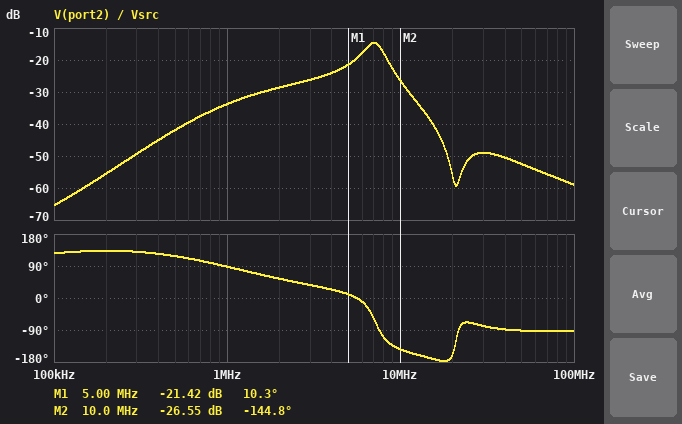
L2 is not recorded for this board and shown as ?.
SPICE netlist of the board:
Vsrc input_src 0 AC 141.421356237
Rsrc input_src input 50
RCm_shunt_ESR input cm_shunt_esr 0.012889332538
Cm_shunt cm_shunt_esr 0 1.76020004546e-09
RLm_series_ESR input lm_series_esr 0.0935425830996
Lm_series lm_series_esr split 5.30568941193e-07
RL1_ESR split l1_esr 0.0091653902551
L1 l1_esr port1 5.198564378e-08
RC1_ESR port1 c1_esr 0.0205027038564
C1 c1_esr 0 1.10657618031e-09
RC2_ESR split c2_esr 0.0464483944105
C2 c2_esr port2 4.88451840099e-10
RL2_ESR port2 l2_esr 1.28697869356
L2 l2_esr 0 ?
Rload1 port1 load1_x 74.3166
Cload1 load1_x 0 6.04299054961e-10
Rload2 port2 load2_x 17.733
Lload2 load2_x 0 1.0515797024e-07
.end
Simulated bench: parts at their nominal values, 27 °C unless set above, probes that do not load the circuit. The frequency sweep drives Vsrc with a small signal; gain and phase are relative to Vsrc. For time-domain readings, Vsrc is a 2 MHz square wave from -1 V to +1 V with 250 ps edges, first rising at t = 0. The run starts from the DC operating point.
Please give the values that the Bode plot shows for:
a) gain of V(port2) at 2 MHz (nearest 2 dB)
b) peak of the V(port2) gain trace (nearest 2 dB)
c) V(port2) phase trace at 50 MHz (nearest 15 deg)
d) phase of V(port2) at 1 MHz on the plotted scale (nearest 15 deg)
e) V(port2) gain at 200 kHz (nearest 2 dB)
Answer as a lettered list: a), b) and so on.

a) -28 dB
b) -14 dB
c) -90 deg
d) 90 deg
e) -56 dB
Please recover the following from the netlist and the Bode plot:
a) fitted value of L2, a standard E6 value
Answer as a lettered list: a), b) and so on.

a) 2.2 µH
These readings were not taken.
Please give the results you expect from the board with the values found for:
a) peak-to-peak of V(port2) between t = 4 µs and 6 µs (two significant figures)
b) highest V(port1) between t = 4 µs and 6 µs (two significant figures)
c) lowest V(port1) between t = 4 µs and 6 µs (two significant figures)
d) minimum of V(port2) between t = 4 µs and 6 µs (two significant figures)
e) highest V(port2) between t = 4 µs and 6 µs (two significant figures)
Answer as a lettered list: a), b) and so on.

a) 220 mV
b) 620 mV
c) -620 mV
d) -110 mV
e) 110 mV
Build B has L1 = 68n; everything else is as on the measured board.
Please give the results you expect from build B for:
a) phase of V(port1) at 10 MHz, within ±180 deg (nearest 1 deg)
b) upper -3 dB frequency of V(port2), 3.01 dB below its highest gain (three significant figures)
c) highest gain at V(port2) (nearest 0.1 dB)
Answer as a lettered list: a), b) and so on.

a) 127 deg
b) 7.85 MHz
c) -14.8 dB
